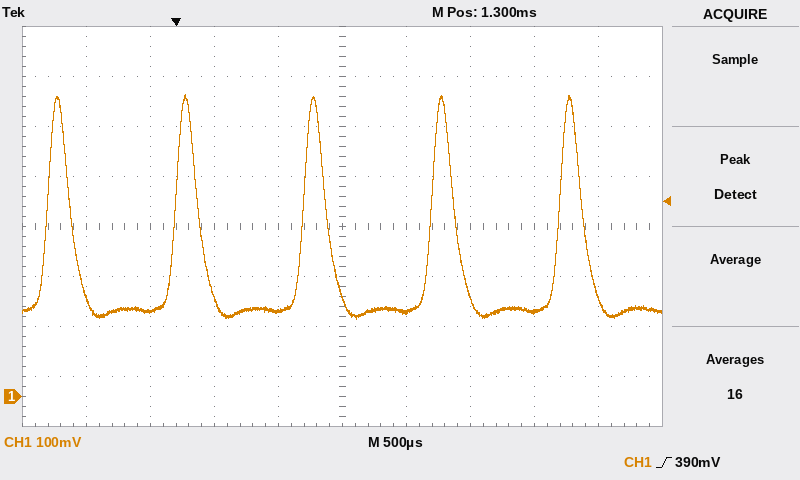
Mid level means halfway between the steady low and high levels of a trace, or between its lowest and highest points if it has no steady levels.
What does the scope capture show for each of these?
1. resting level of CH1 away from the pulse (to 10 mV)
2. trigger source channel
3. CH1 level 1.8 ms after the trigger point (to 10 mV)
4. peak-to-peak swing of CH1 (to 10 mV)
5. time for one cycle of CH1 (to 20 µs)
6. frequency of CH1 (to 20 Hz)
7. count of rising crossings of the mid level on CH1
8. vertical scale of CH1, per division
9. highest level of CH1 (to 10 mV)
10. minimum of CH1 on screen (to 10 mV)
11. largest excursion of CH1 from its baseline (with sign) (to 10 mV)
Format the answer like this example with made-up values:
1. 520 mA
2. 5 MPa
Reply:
1. 170 mV
2. CH1
3. 170 mV
4. 450 mV
5. 1.00 ms
6. 1.00 kHz
7. 5
8. 100 mV
9. 600 mV
10. 150 mV
11. +430 mV
